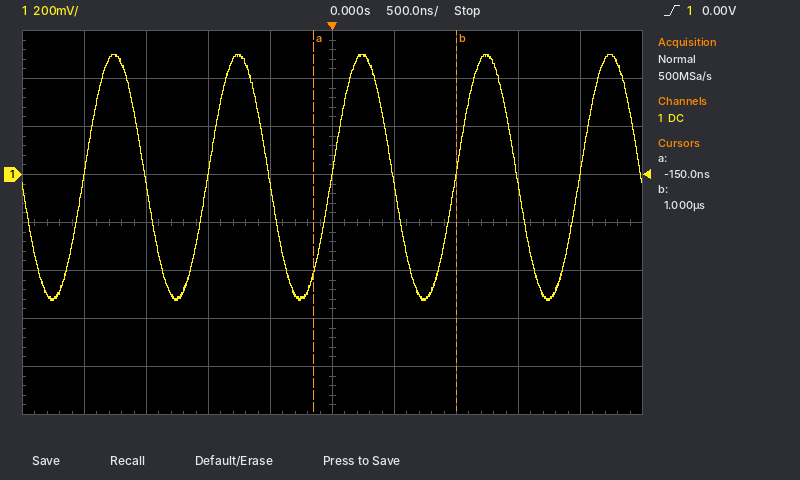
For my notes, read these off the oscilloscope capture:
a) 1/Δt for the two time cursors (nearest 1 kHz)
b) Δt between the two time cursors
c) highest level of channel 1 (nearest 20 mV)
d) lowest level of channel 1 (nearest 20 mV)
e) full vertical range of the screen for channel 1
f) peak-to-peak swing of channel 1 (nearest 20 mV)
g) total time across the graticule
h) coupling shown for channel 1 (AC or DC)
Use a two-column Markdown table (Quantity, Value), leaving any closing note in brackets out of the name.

| Quantity | Value |
|---|---|
| 1/Δt for the two time cursors | 870 kHz |
| Δt between the two time cursors | 1.15 µs |
| highest level of channel 1 | 500 mV |
| lowest level of channel 1 | -520 mV |
| full vertical range of the screen for channel 1 | 1.6 V |
| peak-to-peak swing of channel 1 | 1.02 V |
| total time across the graticule | 5 µs |
| coupling shown for channel 1 | DC |
